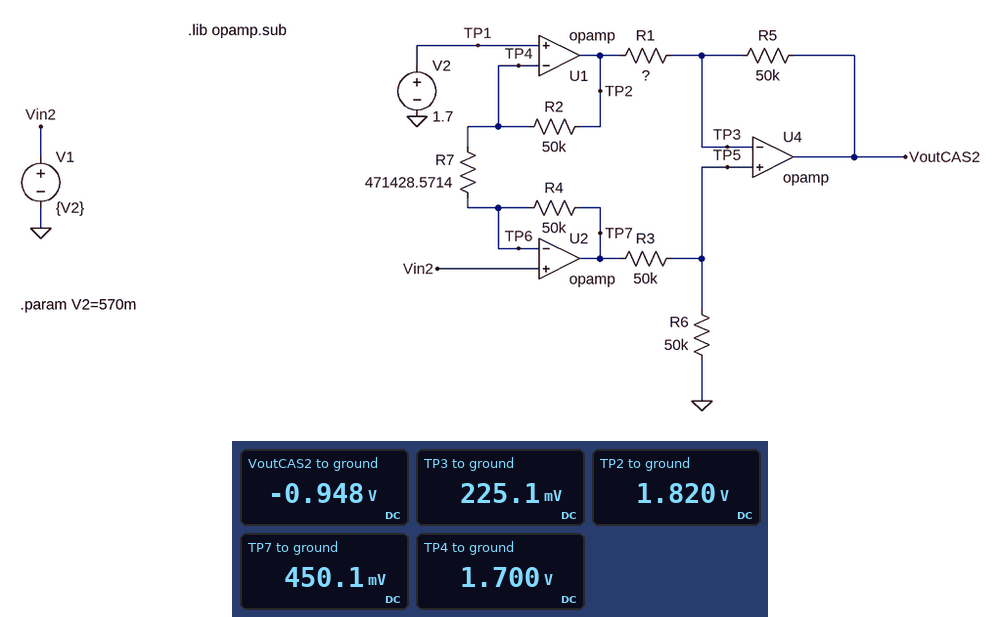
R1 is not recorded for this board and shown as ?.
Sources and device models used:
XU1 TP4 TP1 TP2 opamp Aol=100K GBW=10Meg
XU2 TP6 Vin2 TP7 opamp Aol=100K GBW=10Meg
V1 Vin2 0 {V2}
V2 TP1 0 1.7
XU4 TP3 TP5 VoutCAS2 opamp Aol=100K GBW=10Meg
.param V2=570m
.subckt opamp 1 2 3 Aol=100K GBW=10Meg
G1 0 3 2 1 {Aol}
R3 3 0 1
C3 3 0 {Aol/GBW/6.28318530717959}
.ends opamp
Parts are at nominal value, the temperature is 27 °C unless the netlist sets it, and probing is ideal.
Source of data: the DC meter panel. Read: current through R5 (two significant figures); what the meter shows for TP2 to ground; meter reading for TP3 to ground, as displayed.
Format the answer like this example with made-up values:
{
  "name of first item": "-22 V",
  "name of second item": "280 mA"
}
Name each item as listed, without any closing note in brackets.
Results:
{
  "current through R5": "23 µA",
  "what the meter shows for TP2 to ground": "1.820 V",
  "meter reading for TP3 to ground, as displayed": "225.1 mV"
}
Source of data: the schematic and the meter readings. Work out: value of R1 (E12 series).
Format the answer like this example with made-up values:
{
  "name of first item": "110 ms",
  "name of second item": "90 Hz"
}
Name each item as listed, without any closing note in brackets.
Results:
{
  "value of R1": "68 kΩ"
}
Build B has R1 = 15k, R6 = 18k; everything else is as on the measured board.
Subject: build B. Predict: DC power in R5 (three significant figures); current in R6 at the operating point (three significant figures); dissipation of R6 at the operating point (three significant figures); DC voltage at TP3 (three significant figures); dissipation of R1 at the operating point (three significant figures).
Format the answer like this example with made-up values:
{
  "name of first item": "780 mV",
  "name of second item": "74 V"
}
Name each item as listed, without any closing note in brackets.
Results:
{
  "DC power in R5": "643 µW",
  "current in R6 at the operating point": "6.62 µA",
  "dissipation of R6 at the operating point": "789 nW",
  "DC voltage at TP3": "119 mV",
  "dissipation of R1 at the operating point": "193 µW"
}
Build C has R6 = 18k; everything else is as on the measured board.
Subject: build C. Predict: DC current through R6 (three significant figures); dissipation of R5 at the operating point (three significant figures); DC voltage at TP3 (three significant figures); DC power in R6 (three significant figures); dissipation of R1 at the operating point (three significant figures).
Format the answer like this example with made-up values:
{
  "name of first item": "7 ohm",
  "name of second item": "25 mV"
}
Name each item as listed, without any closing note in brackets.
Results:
{
  "DC current through R6": "6.62 µA",
  "dissipation of R5 at the operating point": "31.3 µW",
  "DC voltage at TP3": "119 mV",
  "DC power in R6": "789 nW",
  "dissipation of R1 at the operating point": "42.5 µW"
}
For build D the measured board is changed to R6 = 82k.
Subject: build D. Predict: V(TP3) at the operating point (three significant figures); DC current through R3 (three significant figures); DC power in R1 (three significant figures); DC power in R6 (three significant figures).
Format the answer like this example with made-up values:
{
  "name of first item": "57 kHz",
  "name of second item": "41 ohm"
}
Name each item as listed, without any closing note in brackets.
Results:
{
  "V(TP3) at the operating point": "280 mV",
  "DC current through R3": "3.41 µA",
  "DC power in R1": "34.9 µW",
  "DC power in R6": "954 nW"
}
